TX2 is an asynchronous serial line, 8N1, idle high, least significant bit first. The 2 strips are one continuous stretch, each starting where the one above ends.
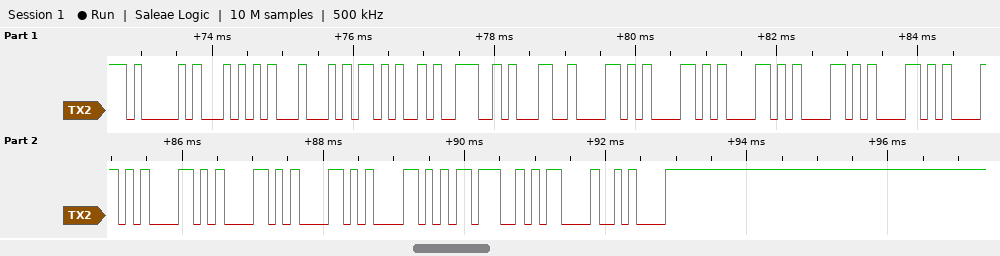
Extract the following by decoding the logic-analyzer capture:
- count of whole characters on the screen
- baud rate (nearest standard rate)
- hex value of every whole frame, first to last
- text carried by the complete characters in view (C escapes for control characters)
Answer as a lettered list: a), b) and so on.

a) 19
b) 9600 baud
c) 41 54 44 2B 39 31 58 58 58 58 58 58 58 58 58 58 3B 0D 0A
d) "ATD+91XXXXXXXXXX;\r\n"
